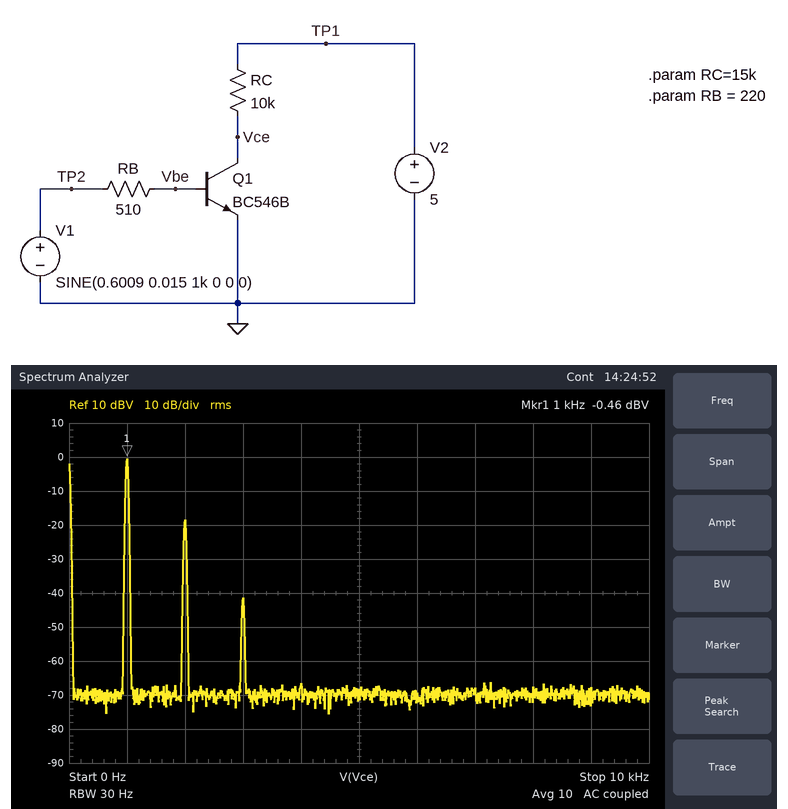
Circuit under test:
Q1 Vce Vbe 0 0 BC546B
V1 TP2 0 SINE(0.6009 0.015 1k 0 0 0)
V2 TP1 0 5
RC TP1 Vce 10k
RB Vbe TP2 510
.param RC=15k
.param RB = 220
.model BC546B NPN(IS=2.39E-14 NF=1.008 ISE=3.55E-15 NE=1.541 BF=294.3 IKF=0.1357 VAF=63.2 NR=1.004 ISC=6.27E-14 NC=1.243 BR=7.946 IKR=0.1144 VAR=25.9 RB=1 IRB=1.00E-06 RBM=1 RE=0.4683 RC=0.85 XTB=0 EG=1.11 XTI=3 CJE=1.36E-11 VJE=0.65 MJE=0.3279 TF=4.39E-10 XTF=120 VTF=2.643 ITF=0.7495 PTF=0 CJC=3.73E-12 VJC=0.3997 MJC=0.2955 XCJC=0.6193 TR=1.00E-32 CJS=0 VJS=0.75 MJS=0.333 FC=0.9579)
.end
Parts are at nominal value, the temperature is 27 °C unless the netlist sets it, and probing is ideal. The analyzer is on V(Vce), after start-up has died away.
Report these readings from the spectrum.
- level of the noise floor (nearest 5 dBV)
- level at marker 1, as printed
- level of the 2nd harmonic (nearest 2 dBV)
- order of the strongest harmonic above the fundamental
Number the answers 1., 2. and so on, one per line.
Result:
1. -70 dBV
2. -0.46 dBV
3. -18 dBV
4. 2
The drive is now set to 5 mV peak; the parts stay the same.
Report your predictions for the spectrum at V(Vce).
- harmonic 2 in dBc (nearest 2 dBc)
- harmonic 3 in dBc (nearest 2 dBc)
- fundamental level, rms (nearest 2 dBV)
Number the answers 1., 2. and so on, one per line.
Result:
1. -28 dBc
2. -60 dBc
3. -10 dBV
